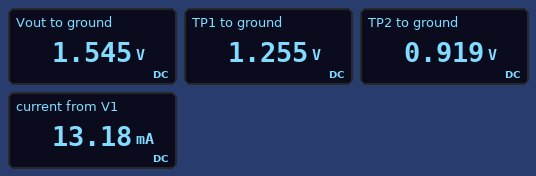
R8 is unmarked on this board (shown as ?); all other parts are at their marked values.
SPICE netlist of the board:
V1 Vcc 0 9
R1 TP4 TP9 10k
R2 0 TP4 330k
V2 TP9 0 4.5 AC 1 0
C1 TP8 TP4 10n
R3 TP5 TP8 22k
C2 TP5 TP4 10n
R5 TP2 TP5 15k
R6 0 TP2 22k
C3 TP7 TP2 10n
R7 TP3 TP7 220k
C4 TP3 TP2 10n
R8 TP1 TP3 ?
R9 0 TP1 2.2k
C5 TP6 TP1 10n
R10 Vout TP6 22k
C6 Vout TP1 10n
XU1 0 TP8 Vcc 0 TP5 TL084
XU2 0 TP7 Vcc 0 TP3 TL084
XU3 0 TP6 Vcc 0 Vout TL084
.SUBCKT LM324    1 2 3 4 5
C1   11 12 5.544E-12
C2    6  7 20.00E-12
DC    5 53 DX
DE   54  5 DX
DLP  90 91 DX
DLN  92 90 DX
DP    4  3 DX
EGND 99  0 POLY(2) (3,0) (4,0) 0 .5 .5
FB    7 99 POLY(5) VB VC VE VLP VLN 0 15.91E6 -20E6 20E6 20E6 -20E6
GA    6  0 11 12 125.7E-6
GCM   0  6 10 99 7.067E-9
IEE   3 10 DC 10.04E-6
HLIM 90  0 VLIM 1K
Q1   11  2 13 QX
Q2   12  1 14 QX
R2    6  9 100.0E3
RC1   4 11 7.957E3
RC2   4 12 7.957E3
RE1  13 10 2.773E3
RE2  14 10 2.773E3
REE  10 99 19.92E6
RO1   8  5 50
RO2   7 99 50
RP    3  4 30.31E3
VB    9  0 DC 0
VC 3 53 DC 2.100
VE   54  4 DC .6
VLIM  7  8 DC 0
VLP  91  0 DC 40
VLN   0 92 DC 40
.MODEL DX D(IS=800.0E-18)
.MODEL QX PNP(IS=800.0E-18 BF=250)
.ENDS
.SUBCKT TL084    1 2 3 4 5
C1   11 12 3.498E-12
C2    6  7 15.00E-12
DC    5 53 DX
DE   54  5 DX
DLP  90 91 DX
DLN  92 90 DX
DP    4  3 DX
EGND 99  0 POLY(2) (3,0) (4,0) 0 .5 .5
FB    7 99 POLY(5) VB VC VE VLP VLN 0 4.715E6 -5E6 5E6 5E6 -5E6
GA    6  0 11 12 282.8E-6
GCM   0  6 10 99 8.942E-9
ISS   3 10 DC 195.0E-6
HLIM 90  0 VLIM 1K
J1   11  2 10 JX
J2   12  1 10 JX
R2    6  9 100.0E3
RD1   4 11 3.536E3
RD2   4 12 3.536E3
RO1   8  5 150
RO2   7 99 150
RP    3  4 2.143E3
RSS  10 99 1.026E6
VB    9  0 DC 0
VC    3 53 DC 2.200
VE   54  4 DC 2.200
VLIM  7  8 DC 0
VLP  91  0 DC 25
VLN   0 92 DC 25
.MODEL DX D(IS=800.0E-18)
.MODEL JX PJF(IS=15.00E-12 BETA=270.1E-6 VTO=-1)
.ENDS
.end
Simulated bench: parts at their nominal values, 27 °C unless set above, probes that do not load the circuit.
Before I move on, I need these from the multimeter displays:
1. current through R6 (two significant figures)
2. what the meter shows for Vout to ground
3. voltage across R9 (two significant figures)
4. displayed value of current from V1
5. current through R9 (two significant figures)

42 µA
1.545 V
1.3 V
13.18 mA
570 µA
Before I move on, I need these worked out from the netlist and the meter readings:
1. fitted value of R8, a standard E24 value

510 Ω
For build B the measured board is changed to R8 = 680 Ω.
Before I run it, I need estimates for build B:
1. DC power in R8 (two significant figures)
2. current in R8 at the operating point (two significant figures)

200 µW
540 µA
